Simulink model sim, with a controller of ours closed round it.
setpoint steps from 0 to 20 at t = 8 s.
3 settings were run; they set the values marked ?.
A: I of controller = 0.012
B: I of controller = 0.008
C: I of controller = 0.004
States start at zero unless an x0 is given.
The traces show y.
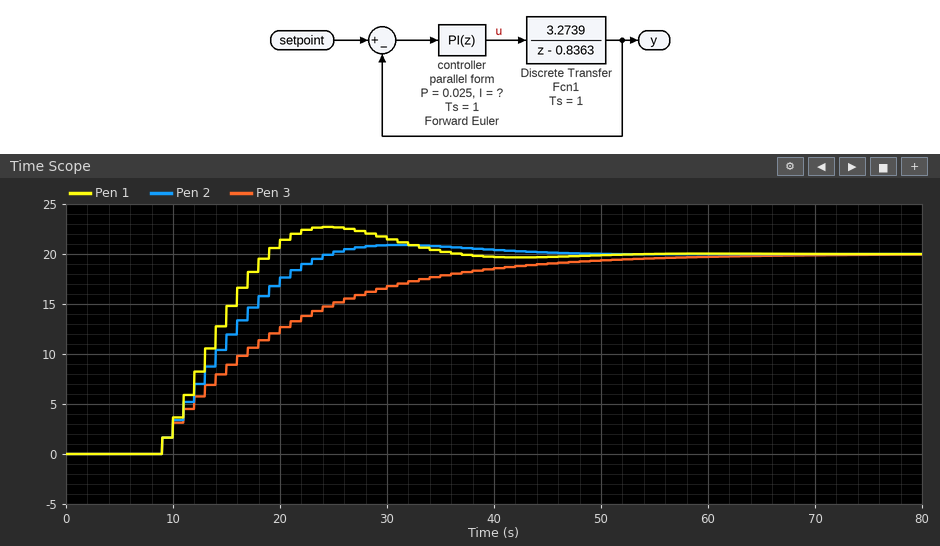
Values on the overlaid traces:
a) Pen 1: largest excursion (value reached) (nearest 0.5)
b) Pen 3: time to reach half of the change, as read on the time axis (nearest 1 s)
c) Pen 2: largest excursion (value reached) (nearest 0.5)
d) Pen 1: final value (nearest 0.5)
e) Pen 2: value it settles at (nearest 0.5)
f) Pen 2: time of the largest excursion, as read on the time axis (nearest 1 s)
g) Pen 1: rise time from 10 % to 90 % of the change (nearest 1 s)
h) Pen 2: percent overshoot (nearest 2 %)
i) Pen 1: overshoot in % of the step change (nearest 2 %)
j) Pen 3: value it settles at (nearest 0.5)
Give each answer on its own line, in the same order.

22.5
17 s
21.0
20.0
20.0
31 s
7 s
4 %
14 %
20.0
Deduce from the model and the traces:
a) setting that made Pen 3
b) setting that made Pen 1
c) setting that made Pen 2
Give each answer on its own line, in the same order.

C
A
B
